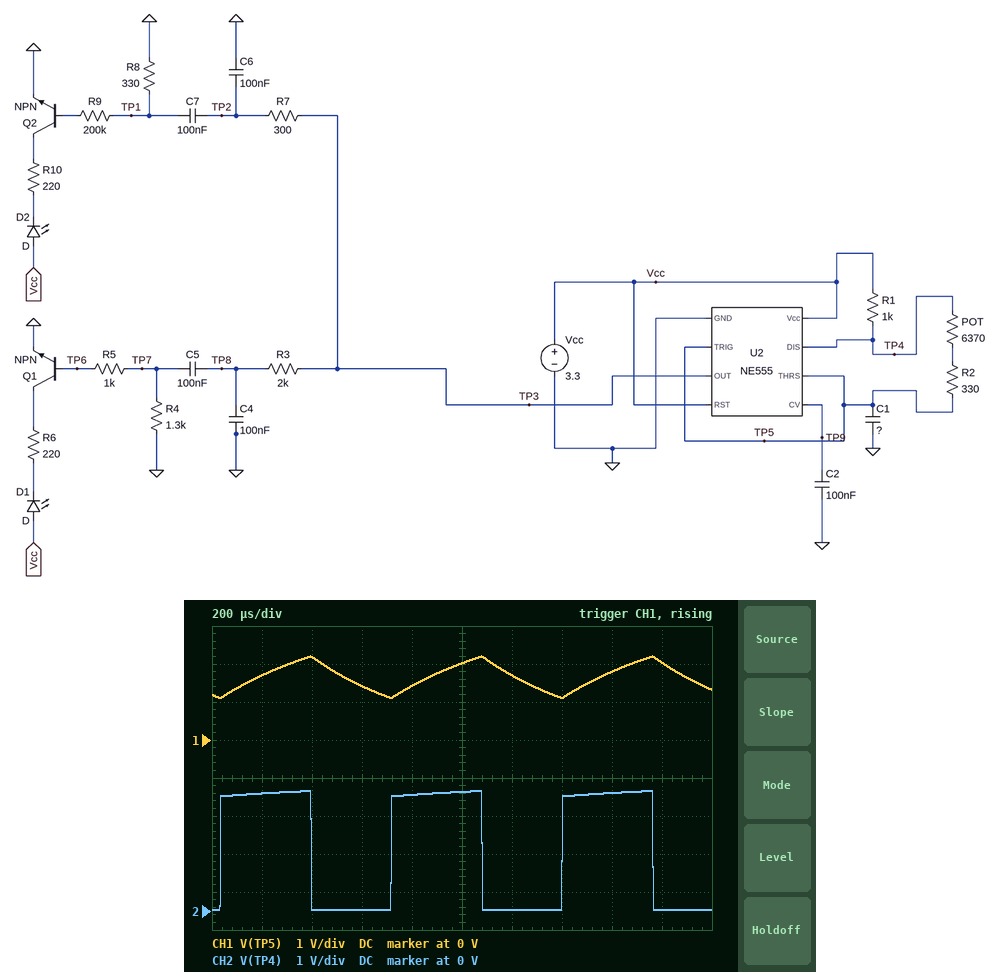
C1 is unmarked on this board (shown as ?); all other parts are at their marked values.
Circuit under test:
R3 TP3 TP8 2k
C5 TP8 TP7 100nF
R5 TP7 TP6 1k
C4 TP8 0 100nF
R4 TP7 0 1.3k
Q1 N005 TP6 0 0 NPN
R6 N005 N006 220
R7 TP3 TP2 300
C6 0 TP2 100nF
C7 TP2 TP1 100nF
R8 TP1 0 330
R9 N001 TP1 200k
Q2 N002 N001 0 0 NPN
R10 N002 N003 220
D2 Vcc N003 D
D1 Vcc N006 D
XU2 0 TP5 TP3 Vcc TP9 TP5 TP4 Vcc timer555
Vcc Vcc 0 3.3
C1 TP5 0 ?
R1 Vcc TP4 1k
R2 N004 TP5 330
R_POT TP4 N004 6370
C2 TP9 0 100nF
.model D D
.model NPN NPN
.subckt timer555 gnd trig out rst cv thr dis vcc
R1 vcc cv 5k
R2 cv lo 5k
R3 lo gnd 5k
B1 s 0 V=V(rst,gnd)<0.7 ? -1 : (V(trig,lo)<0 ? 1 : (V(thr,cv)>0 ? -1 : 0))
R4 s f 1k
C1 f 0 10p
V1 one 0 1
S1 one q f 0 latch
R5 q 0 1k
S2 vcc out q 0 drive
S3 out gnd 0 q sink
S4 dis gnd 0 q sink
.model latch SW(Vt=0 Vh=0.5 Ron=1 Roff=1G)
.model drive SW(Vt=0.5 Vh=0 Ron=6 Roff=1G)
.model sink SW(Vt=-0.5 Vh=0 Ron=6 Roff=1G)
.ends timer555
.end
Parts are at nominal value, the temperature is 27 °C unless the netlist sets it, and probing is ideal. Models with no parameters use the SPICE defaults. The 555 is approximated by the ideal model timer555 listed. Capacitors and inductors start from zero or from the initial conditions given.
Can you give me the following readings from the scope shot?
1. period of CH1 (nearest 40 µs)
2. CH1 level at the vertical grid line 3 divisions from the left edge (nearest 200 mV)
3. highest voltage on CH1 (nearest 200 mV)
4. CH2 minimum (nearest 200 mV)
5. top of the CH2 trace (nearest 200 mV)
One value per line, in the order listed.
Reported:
680 µs
1.4 V
2.2 V
0 V
3.2 V
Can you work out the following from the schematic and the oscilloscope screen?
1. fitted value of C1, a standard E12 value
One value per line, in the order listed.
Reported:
68 nF
